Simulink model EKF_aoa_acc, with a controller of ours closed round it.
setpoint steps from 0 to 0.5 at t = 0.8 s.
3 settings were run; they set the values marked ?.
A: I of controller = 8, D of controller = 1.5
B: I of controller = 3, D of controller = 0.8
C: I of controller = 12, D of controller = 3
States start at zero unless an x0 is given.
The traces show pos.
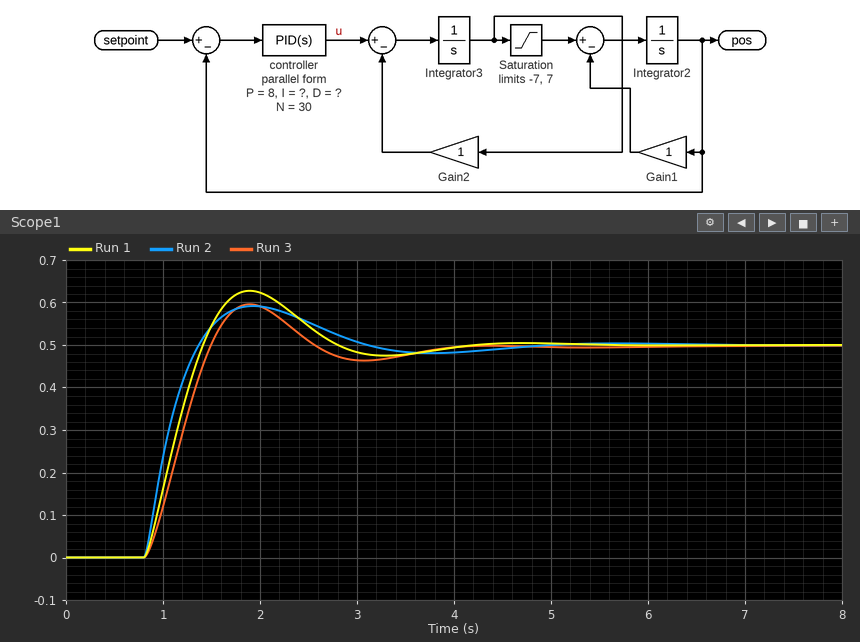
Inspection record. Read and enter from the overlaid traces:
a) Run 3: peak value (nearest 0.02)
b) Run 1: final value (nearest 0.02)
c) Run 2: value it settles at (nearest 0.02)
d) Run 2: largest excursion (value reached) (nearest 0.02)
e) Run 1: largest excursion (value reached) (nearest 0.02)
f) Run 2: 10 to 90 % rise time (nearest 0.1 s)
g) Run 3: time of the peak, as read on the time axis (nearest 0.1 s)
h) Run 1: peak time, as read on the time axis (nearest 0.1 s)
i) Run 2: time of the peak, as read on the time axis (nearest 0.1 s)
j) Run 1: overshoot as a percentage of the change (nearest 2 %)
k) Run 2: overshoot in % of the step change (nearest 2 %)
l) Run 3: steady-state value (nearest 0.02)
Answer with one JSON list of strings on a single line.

["0.60", "0.50", "0.50", "0.60", "0.62", "0.4 s", "1.9 s", "1.9 s", "1.9 s", "26 %", "18 %", "0.50"]
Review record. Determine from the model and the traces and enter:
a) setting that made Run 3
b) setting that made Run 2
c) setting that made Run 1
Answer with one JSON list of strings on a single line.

["B", "C", "A"]
